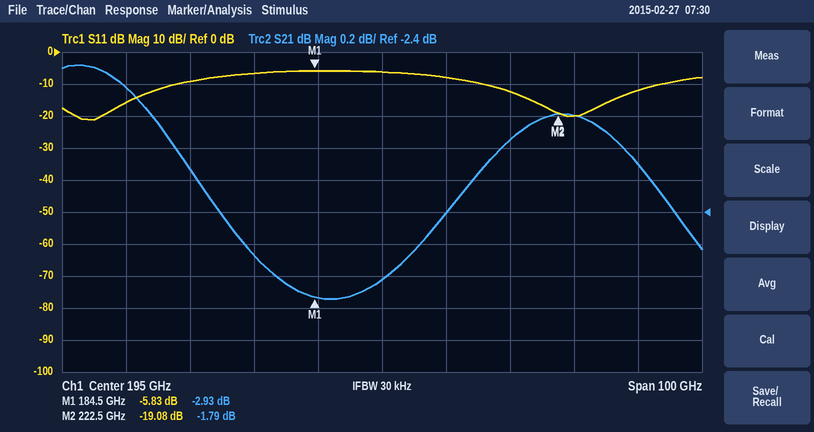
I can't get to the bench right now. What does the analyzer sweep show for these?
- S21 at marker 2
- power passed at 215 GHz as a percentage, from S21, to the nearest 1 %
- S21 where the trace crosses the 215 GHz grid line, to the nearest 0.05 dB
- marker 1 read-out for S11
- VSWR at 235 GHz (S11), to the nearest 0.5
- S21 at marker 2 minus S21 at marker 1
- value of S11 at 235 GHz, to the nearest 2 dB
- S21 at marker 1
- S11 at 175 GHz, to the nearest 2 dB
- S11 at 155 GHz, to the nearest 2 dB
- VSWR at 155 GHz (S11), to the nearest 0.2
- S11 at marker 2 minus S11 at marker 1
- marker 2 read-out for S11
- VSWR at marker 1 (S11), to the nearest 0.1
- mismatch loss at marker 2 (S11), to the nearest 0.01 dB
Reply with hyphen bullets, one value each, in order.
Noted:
- -1.79 dB
- 64 %
- -1.95 dB
- -5.83 dB
- 1.5
- 1.14 dB
- -12 dB
- -2.93 dB
- -6 dB
- -16 dB
- 1.4
- -13.25 dB
- -19.08 dB
- 3.1
- 0.05 dB
